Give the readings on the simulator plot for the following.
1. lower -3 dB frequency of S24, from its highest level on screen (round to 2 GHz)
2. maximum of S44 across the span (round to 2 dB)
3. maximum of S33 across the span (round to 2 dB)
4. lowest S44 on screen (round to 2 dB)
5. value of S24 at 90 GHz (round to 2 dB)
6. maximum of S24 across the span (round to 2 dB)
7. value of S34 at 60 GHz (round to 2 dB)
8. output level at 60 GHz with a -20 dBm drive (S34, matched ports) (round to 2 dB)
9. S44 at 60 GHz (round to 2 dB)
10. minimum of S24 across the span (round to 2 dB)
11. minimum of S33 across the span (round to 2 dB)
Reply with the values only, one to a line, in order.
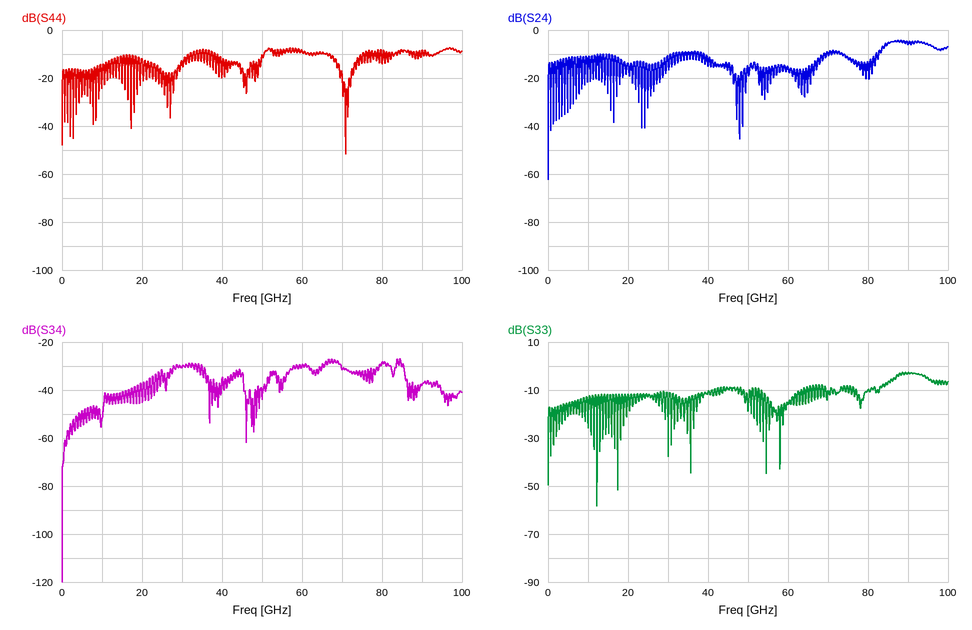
84 GHz
-8 dB
-2 dB
-52 dB
-6 dB
-4 dB
-30 dB
-50 dBm
-8 dB
-62 dB
-58 dB
